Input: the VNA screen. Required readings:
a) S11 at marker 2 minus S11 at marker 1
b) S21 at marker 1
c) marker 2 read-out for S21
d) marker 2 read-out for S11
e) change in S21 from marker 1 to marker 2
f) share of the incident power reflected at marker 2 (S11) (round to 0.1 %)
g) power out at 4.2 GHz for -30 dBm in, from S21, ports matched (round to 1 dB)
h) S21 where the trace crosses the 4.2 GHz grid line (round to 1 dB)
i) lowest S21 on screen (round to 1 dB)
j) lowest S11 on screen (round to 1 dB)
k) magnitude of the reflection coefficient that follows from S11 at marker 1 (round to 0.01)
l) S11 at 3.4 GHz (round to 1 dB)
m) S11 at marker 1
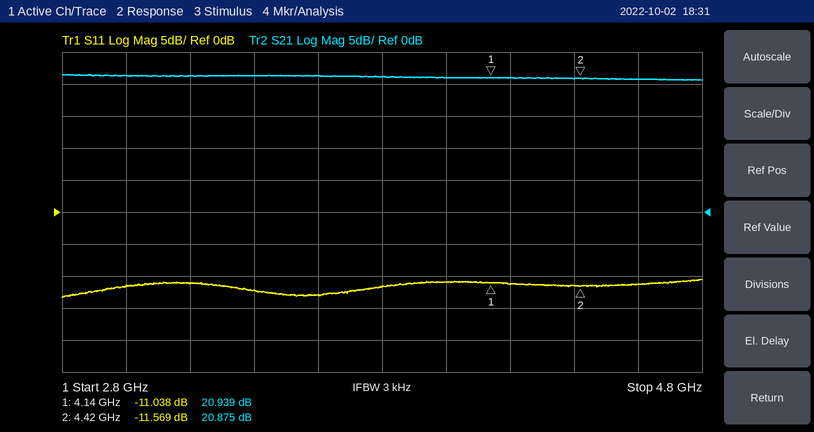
-0.531 dB
20.939 dB
20.875 dB
-11.569 dB
-0.064 dB
7.0 %
-9 dBm
21 dB
21 dB
-13 dB
0.28
-12 dB
-11.038 dB
